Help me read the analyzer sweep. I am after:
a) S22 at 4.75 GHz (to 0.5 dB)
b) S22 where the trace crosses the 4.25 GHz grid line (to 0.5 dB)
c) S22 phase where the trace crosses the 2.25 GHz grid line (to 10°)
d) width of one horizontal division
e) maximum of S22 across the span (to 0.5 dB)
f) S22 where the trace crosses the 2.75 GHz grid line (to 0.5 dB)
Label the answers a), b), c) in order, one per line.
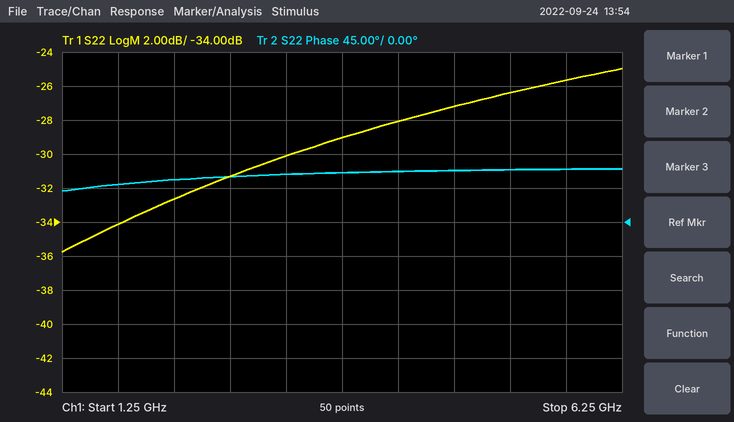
a) -27.0 dB
b) -28.0 dB
c) 60°
d) 500 MHz
e) -25.0 dB
f) -31.5 dB
